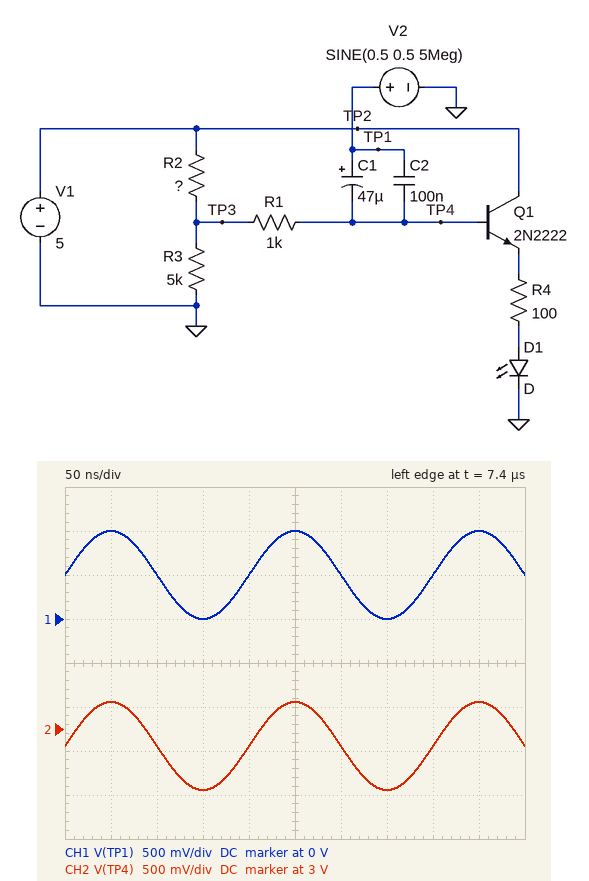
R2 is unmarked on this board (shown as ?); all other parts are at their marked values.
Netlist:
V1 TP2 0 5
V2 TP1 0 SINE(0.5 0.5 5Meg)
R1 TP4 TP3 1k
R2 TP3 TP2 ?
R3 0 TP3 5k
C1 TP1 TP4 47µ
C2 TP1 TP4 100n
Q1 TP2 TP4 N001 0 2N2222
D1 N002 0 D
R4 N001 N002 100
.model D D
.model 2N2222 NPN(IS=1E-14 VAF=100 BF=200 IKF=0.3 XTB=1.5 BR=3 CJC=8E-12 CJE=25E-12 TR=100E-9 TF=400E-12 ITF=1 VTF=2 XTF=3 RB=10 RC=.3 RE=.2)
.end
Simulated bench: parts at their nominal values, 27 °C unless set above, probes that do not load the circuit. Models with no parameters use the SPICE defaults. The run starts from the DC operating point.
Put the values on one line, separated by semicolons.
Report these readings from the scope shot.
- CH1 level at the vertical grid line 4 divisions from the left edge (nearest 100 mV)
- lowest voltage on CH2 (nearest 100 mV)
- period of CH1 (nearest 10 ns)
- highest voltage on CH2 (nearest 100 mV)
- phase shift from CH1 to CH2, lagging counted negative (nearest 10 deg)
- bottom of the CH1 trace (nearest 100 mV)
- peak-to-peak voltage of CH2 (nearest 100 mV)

500 mV; 2.3 V; 200 ns; 3.3 V; 0 deg; 0 V; 1.0 V
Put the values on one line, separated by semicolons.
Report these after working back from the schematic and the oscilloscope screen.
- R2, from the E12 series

3.3 kΩ
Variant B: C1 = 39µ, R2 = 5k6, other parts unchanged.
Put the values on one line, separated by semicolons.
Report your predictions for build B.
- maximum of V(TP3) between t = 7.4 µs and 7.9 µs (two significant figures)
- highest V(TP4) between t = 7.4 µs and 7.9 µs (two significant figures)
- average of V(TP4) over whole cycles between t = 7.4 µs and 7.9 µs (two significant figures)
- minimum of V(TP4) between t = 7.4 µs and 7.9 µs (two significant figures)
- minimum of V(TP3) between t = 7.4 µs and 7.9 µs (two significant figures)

2.6 V; 2.7 V; 2.2 V; 1.7 V; 1.9 V
